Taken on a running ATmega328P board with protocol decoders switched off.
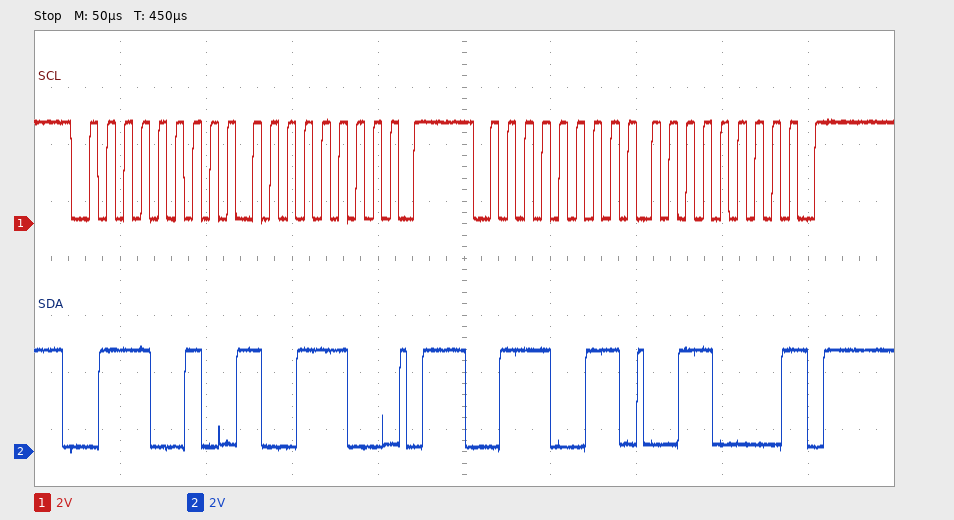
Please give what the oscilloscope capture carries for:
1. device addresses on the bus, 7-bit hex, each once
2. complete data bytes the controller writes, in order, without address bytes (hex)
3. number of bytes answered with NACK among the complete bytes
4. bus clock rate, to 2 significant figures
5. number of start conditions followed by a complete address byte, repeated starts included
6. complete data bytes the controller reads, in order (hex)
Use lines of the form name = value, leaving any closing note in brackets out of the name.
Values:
device addresses on the bus, 7-bit hex, each once = 0x39
complete data bytes the controller writes, in order, without address bytes = 9C
number of bytes answered with NACK among the complete bytes = 1
bus clock rate, to 2 significant figures = 100 kHz
number of start conditions followed by a complete address byte, repeated starts included = 2
complete data bytes the controller reads, in order = 30
